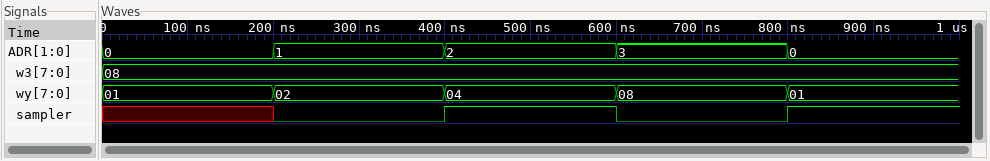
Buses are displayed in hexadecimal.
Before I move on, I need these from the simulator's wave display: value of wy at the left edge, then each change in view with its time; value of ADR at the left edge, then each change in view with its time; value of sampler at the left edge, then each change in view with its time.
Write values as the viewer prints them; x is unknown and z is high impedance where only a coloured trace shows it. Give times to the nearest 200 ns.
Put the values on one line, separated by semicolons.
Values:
01, 02 at 200 ns, 04 at 400 ns, 08 at 600 ns, 01 at 800 ns; 0, 1 at 200 ns, 2 at 400 ns, 3 at 600 ns, 0 at 800 ns; x, 0 at 200 ns, 1 at 400 ns, 0 at 600 ns, 1 at 800 ns
